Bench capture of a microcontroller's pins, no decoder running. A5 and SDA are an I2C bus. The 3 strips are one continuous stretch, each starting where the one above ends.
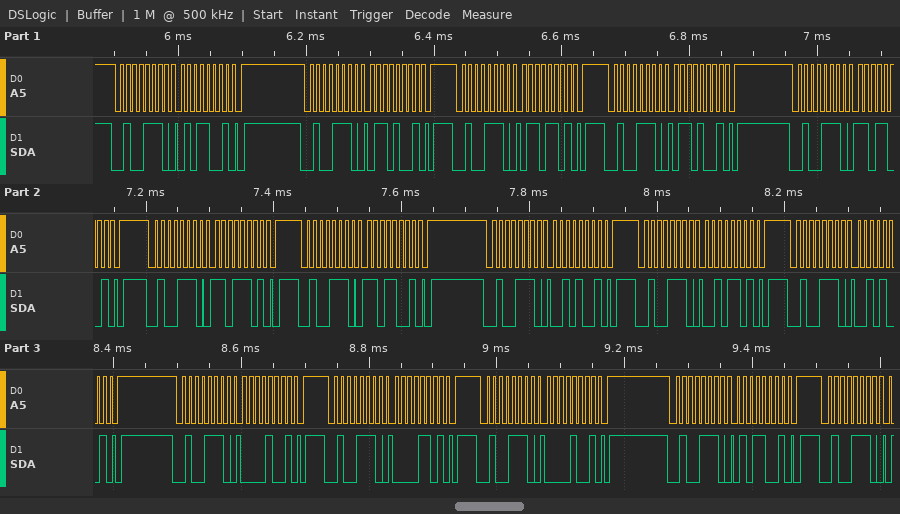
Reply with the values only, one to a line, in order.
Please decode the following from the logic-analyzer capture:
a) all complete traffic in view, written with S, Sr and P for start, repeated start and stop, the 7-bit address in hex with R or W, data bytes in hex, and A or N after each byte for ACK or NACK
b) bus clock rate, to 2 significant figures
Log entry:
S 27W A 59 A P S 27W A 69 A P S 27W A 6D A P S 27W A 69 A P S 27W A D9 A P S 27W A DD A P S 27W A D9 A P S 27W A 29 A P S 27W A 2D A P S 27W A 29 A P S 27W A 09 A P S 27W A 0D A P S 27W A 09 A P S 27W A 59 A P S 27W A
100 kHz
